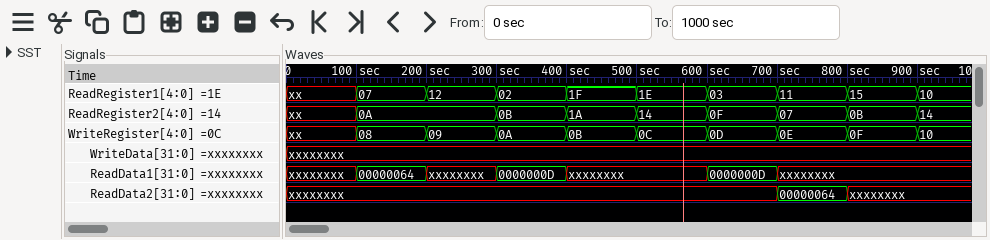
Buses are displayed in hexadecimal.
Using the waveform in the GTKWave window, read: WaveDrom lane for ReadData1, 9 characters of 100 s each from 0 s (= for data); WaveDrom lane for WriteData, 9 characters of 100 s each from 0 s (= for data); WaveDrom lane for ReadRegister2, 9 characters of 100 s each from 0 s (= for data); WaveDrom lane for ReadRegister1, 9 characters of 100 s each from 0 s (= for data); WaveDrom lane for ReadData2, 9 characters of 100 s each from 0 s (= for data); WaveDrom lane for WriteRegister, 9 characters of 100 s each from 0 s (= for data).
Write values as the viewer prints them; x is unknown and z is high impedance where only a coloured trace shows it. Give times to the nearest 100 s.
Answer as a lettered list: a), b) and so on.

a) {name: 'ReadData1', wave: 'x=x=x.=x.', data: '00000064 0000000D 0000000D'}
b) {name: 'WriteData', wave: 'x........'}
c) {name: 'ReadRegister2', wave: 'x=.======', data: '0A 0B 1A 14 0F 07 0B'}
d) {name: 'ReadRegister1', wave: 'x========', data: '07 12 02 1F 1E 03 11 15'}
e) {name: 'ReadData2', wave: 'x......=x', data: '00000064'}
f) {name: 'WriteRegister', wave: 'x========', data: '08 09 0A 0B 0C 0D 0E 0F'}
